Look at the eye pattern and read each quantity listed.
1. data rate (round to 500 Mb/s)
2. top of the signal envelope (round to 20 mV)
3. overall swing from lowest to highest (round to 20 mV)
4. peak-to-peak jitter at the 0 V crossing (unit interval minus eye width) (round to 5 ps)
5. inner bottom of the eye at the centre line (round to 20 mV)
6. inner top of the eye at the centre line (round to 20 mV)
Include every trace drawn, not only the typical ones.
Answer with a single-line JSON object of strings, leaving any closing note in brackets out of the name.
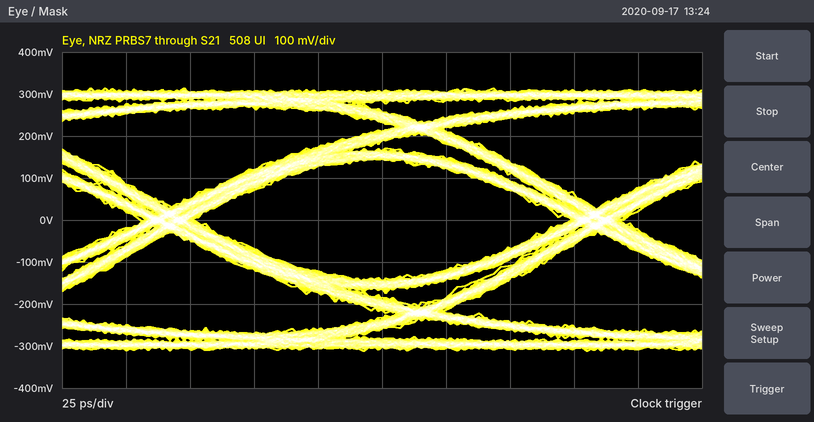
{"data rate": "6.0 Gb/s", "top of the signal envelope": "320 mV", "overall swing from lowest to highest": "620 mV", "peak-to-peak jitter at the 0 V crossing (unit interval minus eye width)": "20 ps", "inner bottom of the eye at the centre line": "-140 mV", "inner top of the eye at the centre line": "140 mV"}
